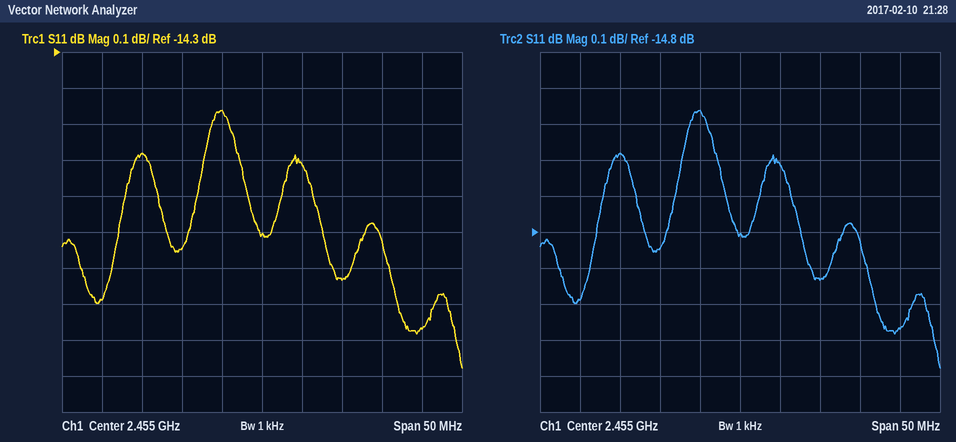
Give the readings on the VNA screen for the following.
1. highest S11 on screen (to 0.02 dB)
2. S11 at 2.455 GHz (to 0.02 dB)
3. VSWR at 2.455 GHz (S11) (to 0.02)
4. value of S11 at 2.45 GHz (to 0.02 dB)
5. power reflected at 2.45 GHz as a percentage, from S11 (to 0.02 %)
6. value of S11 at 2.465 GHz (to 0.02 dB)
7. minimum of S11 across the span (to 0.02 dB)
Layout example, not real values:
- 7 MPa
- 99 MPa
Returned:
- -14.46 dB
- -14.80 dB
- 1.44
- -14.46 dB
- 3.58 %
- -14.94 dB
- -15.18 dB
